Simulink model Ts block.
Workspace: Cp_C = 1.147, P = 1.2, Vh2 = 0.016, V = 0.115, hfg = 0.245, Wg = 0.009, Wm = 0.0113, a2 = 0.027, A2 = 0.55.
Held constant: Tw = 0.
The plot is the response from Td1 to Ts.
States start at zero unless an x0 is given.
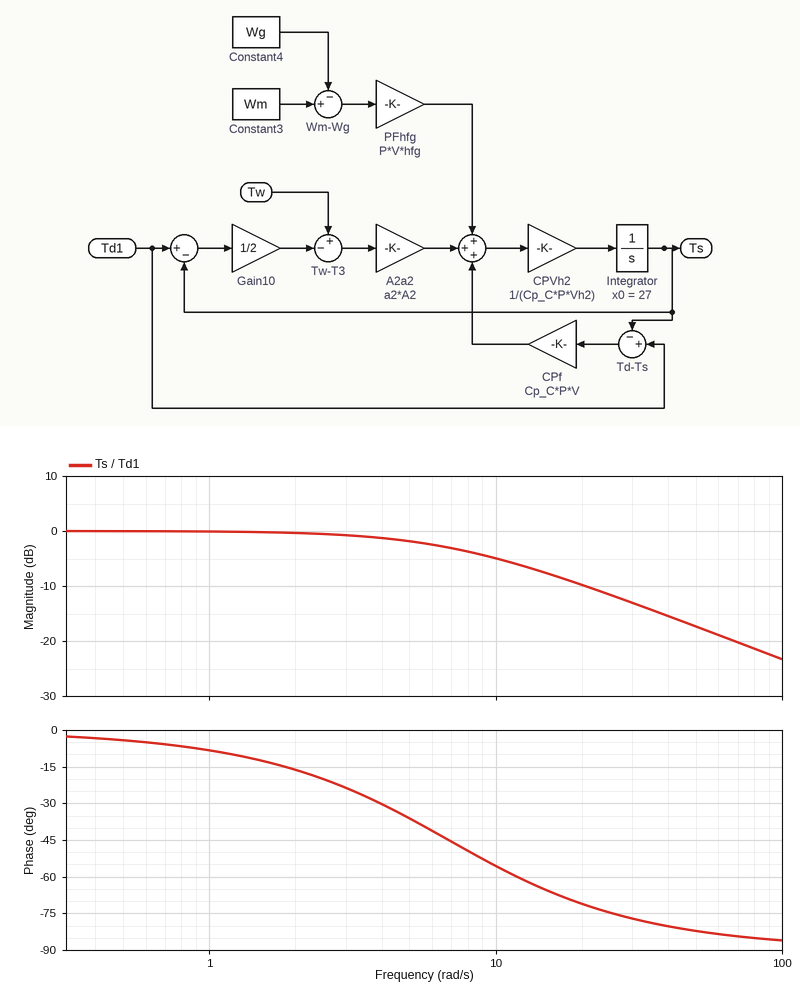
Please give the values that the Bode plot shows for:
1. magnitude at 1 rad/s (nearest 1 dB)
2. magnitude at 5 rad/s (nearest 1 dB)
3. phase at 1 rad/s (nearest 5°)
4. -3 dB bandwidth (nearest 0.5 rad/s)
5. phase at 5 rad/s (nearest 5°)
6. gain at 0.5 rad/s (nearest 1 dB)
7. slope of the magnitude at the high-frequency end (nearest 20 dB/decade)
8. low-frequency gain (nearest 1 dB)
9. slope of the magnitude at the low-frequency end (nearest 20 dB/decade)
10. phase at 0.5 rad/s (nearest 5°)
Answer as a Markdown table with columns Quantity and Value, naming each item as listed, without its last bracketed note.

| Quantity | Value |
|---|---|
| magnitude at 1 rad/s | 0 dB |
| magnitude at 5 rad/s | -2 dB |
| phase at 1 rad/s | -10° |
| -3 dB bandwidth | 7.0 rad/s |
| phase at 5 rad/s | -35° |
| gain at 0.5 rad/s | 0 dB |
| slope of the magnitude at the high-frequency end | -20 dB/decade |
| low-frequency gain | 0 dB |
| slope of the magnitude at the low-frequency end | 0 dB/decade |
| phase at 0.5 rad/s | -5° |
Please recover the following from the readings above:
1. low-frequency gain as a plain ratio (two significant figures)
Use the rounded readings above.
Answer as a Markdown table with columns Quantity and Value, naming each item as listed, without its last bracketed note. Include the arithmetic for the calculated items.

| Quantity | Value |
|---|---|
| low-frequency gain as a plain ratio | 10^(0 / 20) = 1.0 |
